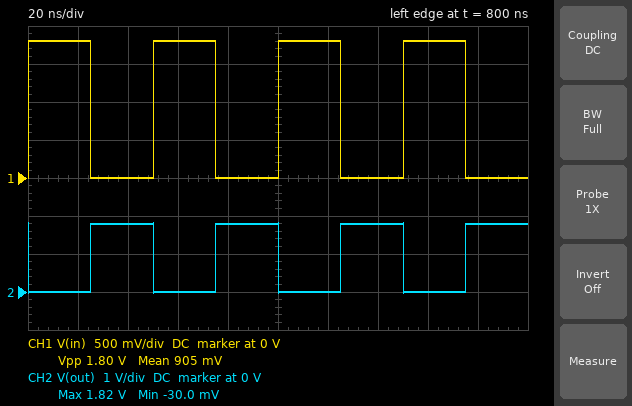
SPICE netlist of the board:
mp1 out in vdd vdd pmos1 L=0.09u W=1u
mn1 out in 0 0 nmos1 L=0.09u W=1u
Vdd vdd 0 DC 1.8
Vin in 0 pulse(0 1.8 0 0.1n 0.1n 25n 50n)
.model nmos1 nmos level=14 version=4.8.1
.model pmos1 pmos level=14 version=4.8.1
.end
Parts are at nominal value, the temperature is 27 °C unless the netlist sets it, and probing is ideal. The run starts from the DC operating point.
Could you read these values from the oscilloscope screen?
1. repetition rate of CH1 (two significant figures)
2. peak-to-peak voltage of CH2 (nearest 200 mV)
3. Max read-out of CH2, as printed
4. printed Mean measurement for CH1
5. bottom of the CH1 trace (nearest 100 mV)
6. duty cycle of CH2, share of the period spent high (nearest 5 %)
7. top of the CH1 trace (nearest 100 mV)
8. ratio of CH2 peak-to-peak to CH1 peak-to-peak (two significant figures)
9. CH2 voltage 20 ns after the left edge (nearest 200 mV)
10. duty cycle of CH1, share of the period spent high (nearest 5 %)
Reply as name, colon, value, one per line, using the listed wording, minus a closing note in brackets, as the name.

repetition rate of CH1: 20 MHz
peak-to-peak voltage of CH2: 1.8 V
Max read-out of CH2, as printed: 1.82 V
printed Mean measurement for CH1: 905 mV
bottom of the CH1 trace: 0 V
duty cycle of CH2, share of the period spent high: 50 %
top of the CH1 trace: 1.8 V
ratio of CH2 peak-to-peak to CH1 peak-to-peak: 1.0
CH2 voltage 20 ns after the left edge: 0 V
duty cycle of CH1, share of the period spent high: 50 %
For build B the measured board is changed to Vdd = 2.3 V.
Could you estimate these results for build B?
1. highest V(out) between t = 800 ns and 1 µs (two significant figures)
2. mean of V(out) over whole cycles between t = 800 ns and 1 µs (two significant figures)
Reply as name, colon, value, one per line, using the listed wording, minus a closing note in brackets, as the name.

highest V(out) between t = 800 ns and 1 µs: 2.3 V
mean of V(out) over whole cycles between t = 800 ns and 1 µs: 1.2 V
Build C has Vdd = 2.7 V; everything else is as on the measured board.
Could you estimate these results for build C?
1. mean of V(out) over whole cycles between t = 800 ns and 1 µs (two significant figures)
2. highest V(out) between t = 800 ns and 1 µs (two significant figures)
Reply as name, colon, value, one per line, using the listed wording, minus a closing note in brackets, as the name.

mean of V(out) over whole cycles between t = 800 ns and 1 µs: 1.4 V
highest V(out) between t = 800 ns and 1 µs: 2.7 V
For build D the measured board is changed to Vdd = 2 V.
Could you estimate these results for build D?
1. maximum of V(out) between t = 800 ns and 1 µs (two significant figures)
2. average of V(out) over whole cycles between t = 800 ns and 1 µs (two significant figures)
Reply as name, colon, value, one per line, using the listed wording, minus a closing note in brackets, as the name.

maximum of V(out) between t = 800 ns and 1 µs: 2.0 V
average of V(out) over whole cycles between t = 800 ns and 1 µs: 1.0 V
